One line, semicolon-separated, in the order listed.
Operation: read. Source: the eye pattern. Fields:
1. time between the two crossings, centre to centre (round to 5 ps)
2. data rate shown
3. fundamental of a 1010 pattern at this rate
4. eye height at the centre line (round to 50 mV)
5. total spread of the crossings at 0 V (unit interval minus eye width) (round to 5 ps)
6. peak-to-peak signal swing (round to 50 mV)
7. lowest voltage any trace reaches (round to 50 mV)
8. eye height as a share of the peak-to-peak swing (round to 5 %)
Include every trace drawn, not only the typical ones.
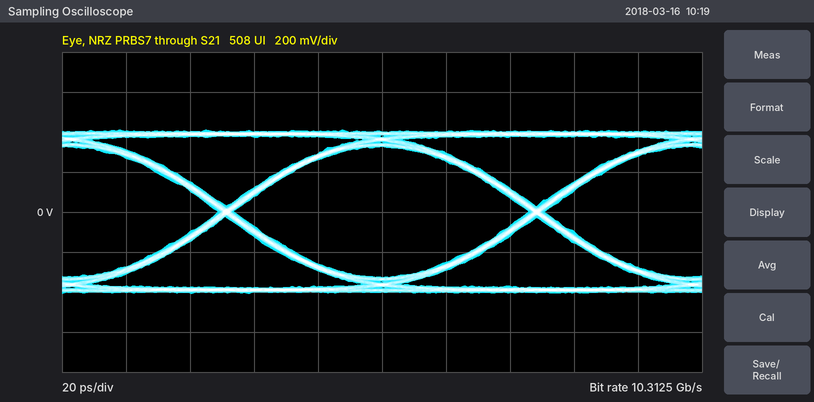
95 ps; 10.3125 Gb/s; 5.15625 GHz; 650 mV; 5 ps; 800 mV; -400 mV; 80 %
